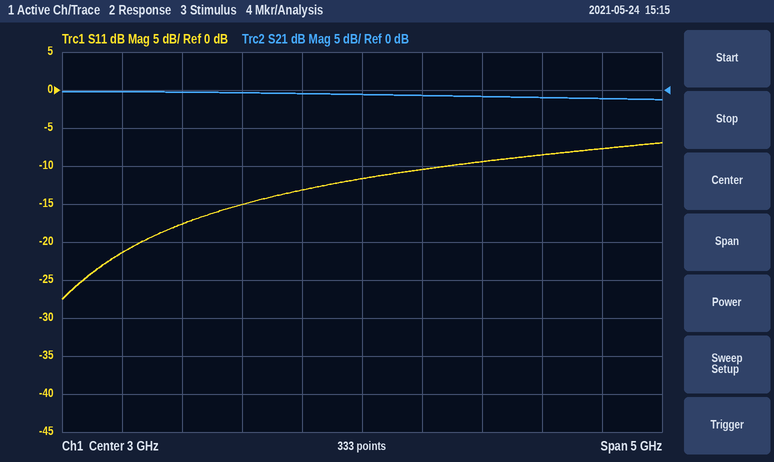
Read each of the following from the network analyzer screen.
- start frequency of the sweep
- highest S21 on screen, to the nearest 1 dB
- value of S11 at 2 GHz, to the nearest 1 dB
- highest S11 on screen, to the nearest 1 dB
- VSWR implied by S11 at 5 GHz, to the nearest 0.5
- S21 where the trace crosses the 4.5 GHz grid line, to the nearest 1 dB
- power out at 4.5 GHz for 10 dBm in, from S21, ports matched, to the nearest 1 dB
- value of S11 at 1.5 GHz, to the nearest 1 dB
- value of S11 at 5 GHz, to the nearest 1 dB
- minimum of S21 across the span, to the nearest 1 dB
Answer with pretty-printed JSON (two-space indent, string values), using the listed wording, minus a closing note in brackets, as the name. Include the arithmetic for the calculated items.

{
  "start frequency of the sweep": "500 MHz",
  "highest S21 on screen, to the nearest 1 dB": "0 dB",
  "value of S11 at 2 GHz, to the nearest 1 dB": "-15 dB",
  "highest S11 on screen, to the nearest 1 dB": "-7 dB",
  "VSWR implied by S11 at 5 GHz, to the nearest 0.5": "|Γ| = 10^(-8/20) = 0.3981; VSWR = (1 + 0.3981)/(1 − 0.3981) ≈ 2.32, so 2.5 to the nearest 0.5",
  "S21 where the trace crosses the 4.5 GHz grid line, to the nearest 1 dB": "-1 dB",
  "power out at 4.5 GHz for 10 dBm in, from S21, ports matched, to the nearest 1 dB": "10 dBm + (-1 dB) = 9 dBm",
  "value of S11 at 1.5 GHz, to the nearest 1 dB": "-18 dB",
  "value of S11 at 5 GHz, to the nearest 1 dB": "-8 dB",
  "minimum of S21 across the span, to the nearest 1 dB": "-1 dB"
}
